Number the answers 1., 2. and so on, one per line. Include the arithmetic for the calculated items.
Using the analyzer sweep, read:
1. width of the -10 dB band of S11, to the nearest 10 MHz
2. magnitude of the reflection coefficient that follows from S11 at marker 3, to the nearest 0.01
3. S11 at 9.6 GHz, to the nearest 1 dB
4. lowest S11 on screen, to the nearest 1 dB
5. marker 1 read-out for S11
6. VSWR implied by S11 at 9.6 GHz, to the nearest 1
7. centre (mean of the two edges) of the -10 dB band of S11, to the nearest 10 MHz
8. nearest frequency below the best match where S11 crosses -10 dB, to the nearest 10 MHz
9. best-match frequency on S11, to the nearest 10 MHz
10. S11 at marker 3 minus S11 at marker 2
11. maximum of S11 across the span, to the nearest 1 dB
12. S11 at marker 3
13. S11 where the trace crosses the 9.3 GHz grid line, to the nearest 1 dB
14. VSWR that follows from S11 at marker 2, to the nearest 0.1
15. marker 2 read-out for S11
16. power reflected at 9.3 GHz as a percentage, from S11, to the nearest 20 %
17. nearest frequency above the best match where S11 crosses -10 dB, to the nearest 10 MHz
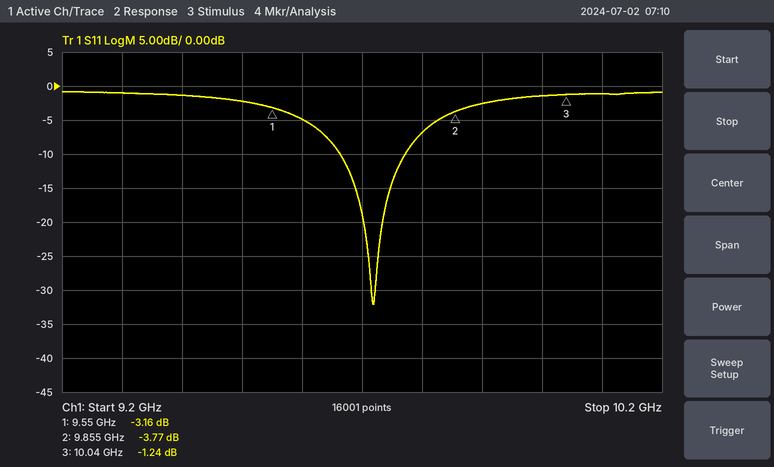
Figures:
1. 9.77 GHz − 9.66 GHz = 110 MHz
2. 10^(-1.24/20) ≈ 0.87
3. -5 dB
4. -32 dB
5. -3.16 dB
6. |Γ| = 10^(-5/20) = 0.5623; VSWR = (1 + 0.5623)/(1 − 0.5623) ≈ 4
7. 9.72 GHz
8. 9.66 GHz
9. 9.72 GHz
10. -1.24 − (-3.77) = 2.53 dB
11. -1 dB
12. -1.24 dB
13. -1 dB
14. (1 + 0.6479)/(1 − 0.6479) ≈ 4.7
15. -3.77 dB
16. 10^(-1/10) ≈ 79.4 %, so 80 % to the nearest 20 %
17. 9.77 GHz
